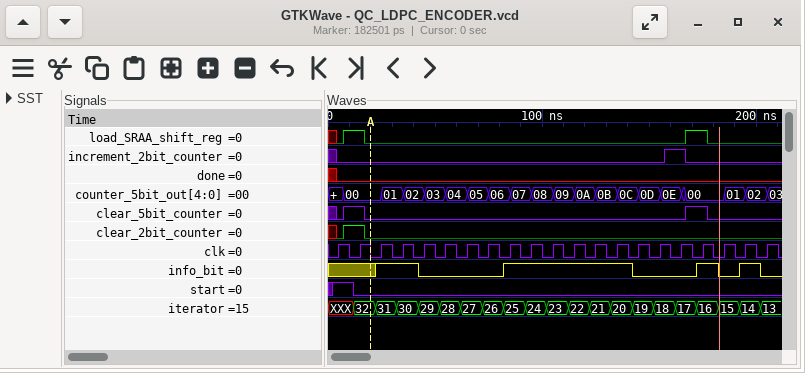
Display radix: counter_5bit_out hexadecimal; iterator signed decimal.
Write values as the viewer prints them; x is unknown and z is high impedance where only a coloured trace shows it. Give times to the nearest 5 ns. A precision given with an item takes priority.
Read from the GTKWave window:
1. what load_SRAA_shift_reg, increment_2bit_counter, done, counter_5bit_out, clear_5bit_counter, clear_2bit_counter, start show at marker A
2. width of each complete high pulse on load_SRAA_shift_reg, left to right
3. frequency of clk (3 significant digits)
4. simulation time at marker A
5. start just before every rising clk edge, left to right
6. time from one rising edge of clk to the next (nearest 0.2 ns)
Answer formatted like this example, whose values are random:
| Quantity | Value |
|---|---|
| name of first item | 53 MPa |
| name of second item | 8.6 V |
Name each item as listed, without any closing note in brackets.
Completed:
| Quantity | Value |
|---|---|
| what load_SRAA_shift_reg, increment_2bit_counter, done, counter_5bit_out, clear_5bit_counter, clear_2bit_counter, start show at marker A | load_SRAA_shift_reg=0, increment_2bit_counter=0, done=0, counter_5bit_out=00, clear_5bit_counter=0, clear_2bit_counter=0, start=0 |
| width of each complete high pulse on load_SRAA_shift_reg, left to right | 10 ns, 10 ns |
| frequency of clk | 100 MHz |
| simulation time at marker A | 20 ns |
| start just before every rising clk edge, left to right | 1 0 0 0 0 0 0 0 0 0 0 0 0 0 0 0 0 0 0 0 0 |
| time from one rising edge of clk to the next | 10 ns |
